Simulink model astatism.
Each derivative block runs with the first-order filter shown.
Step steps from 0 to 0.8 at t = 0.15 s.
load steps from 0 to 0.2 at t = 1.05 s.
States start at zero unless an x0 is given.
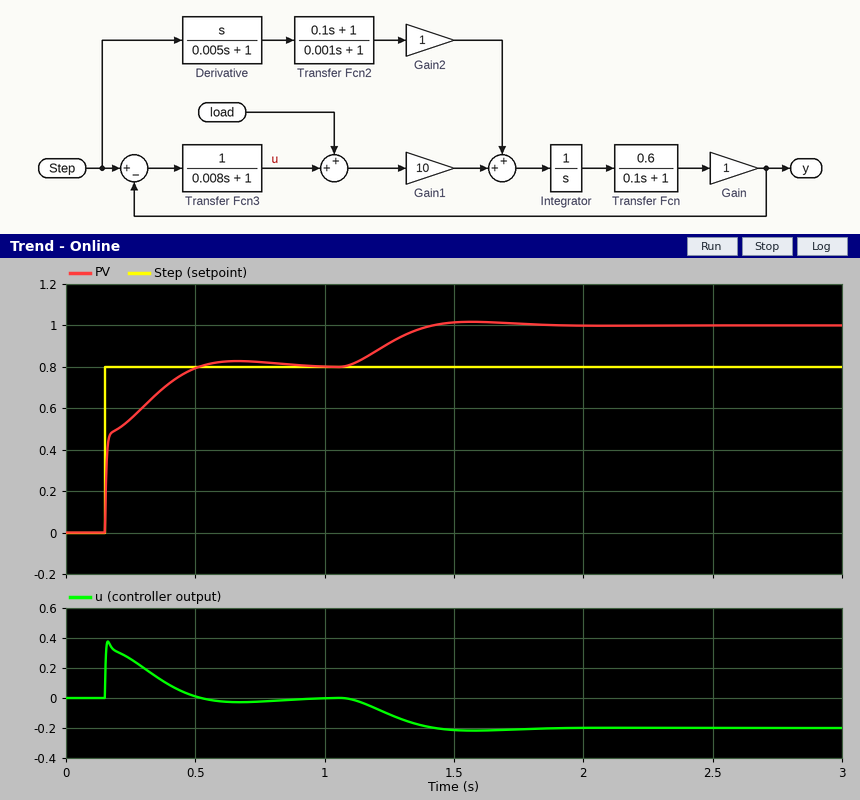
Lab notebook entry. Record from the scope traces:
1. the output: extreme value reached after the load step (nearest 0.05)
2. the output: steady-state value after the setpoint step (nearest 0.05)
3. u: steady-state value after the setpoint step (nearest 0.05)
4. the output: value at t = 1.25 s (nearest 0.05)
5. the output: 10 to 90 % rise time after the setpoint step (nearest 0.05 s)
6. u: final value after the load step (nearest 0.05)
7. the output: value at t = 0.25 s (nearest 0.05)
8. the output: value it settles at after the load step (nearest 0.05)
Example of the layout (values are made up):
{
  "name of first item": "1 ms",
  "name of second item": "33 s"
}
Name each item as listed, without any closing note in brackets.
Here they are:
{
  "the output: extreme value reached after the load step": "1.00",
  "the output: steady-state value after the setpoint step": "0.80",
  "u: steady-state value after the setpoint step": "0.00",
  "the output: value at t = 1.25 s": "0.90",
  "the output: 10 to 90 % rise time after the setpoint step": "0.25 s",
  "u: final value after the load step": "-0.20",
  "the output: value at t = 0.25 s": "0.55",
  "the output: value it settles at after the load step": "1.00"
}
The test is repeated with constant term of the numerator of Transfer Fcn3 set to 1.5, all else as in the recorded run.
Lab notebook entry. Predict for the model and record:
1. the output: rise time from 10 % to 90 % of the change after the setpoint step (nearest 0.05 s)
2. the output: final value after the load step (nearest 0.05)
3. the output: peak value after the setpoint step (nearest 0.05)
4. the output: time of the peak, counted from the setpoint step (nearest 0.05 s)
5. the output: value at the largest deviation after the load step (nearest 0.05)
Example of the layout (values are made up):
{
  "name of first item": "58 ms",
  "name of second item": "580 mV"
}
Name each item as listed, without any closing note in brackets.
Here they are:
{
  "the output: rise time from 10 % to 90 % of the change after the setpoint step": "0.20 s",
  "the output: final value after the load step": "0.95",
  "the output: peak value after the setpoint step": "0.85",
  "the output: time of the peak, counted from the setpoint step": "0.40 s",
  "the output: value at the largest deviation after the load step": "0.95"
}
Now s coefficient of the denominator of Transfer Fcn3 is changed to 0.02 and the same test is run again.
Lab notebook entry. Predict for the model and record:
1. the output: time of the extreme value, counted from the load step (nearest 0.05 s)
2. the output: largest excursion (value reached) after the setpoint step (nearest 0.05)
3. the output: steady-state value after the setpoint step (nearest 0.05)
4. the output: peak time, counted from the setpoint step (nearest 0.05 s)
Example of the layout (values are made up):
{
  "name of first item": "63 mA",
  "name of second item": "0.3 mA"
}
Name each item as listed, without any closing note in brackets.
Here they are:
{
  "the output: time of the extreme value, counted from the load step": "0.50 s",
  "the output: largest excursion (value reached) after the setpoint step": "0.85",
  "the output: steady-state value after the setpoint step": "0.80",
  "the output: peak time, counted from the setpoint step": "0.50 s"
}
